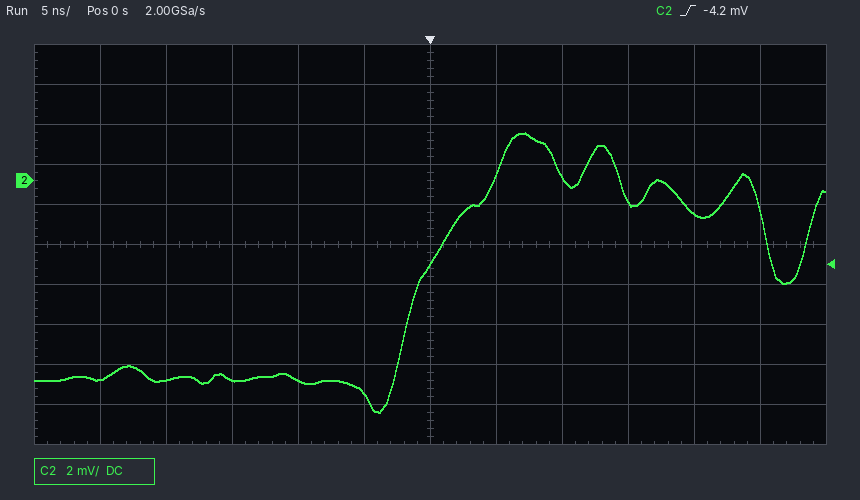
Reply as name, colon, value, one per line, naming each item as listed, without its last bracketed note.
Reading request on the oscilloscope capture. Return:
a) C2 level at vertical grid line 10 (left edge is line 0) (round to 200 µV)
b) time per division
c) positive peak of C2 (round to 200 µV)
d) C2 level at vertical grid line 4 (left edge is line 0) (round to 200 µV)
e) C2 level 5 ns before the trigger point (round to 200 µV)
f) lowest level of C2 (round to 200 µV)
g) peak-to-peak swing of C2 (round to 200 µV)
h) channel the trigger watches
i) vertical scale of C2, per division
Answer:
C2 level at vertical grid line 10 (left edge is line 0): -1.6 mV
time per division: 5 ns
positive peak of C2: 2.4 mV
C2 level at vertical grid line 4 (left edge is line 0): -10.0 mV
C2 level 5 ns before the trigger point: -10.6 mV
lowest level of C2: -11.6 mV
peak-to-peak swing of C2: 14.0 mV
channel the trigger watches: C2
vertical scale of C2, per division: 2 mV
